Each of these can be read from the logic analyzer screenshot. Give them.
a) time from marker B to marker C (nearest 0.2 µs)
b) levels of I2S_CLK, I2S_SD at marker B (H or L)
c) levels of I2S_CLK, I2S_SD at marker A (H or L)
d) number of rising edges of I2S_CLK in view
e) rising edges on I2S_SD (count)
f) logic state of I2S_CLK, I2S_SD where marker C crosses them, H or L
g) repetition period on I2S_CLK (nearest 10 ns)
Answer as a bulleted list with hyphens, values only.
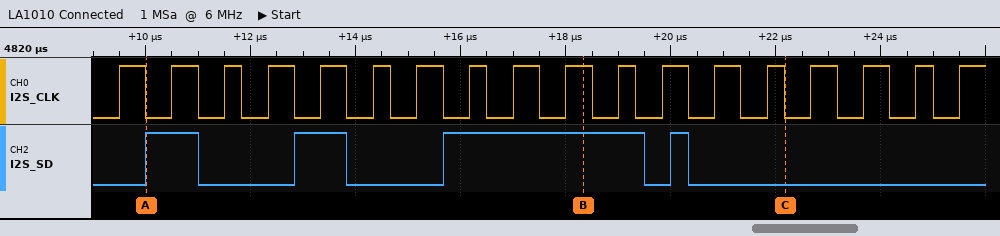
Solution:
- 3.8 µs
- I2S_CLK=H, I2S_SD=H
- I2S_CLK=L, I2S_SD=H
- 18
- 4
- I2S_CLK=L, I2S_SD=L
- 940 ns
